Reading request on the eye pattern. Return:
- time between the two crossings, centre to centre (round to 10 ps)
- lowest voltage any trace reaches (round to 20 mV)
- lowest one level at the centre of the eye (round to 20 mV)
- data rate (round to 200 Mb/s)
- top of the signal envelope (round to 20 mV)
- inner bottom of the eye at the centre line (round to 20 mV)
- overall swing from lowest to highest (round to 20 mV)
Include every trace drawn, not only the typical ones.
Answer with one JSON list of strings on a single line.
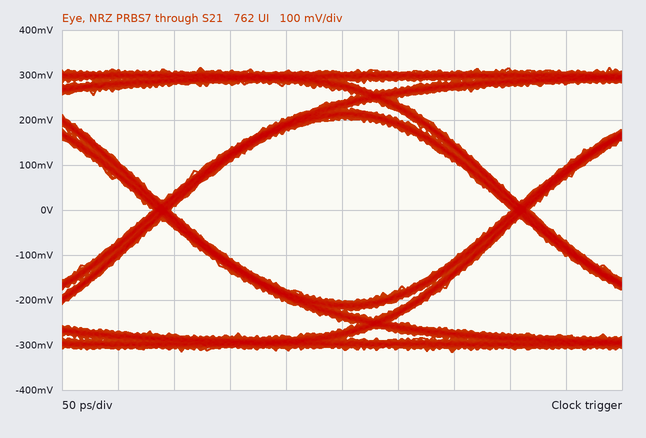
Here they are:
["320 ps", "-320 mV", "200 mV", "3.2 Gb/s", "320 mV", "-200 mV", "640 mV"]
